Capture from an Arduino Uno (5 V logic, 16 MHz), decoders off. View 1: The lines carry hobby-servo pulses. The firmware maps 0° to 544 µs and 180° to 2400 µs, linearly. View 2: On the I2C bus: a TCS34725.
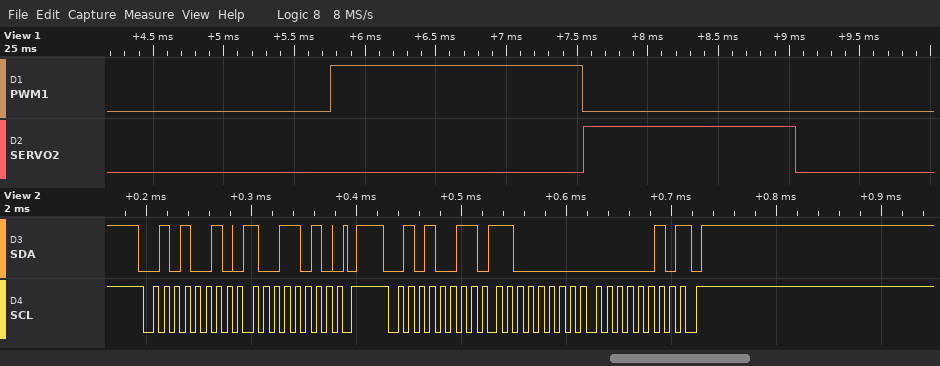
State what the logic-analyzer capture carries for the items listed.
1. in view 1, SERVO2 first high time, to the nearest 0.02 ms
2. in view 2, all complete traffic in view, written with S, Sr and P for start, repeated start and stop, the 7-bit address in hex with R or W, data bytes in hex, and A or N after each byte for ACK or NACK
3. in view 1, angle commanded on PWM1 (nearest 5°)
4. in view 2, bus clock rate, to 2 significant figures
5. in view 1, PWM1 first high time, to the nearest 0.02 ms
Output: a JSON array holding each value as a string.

["1.50 ms", "S 29W A 9A A P S 29R A C0 A 02 N P", "120°", "100 kHz", "1.78 ms"]
